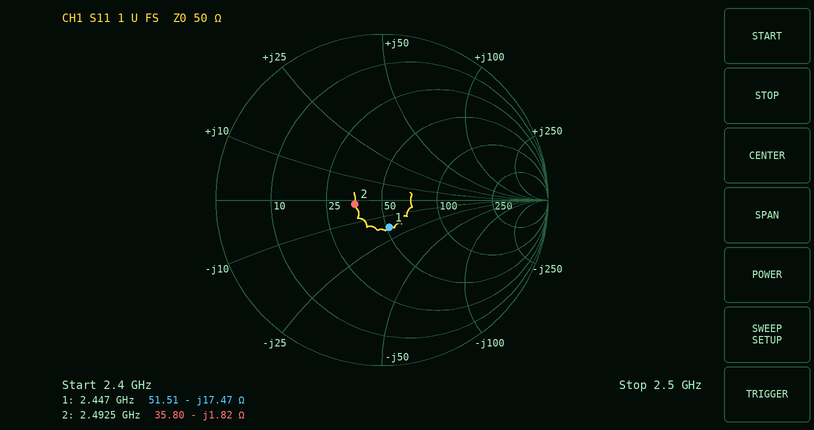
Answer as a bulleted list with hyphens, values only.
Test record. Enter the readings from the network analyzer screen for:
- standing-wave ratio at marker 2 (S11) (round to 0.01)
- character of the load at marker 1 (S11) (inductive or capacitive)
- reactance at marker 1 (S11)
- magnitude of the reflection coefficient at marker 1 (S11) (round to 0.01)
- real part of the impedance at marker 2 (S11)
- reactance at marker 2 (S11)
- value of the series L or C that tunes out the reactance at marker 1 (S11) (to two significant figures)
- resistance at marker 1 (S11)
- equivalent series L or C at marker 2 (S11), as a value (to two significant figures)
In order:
- 1.40
- capacitive
- -17.47 Ω
- 0.17
- 35.80 Ω
- -1.82 Ω
- 1.1 nH
- 51.51 Ω
- 35 pF
